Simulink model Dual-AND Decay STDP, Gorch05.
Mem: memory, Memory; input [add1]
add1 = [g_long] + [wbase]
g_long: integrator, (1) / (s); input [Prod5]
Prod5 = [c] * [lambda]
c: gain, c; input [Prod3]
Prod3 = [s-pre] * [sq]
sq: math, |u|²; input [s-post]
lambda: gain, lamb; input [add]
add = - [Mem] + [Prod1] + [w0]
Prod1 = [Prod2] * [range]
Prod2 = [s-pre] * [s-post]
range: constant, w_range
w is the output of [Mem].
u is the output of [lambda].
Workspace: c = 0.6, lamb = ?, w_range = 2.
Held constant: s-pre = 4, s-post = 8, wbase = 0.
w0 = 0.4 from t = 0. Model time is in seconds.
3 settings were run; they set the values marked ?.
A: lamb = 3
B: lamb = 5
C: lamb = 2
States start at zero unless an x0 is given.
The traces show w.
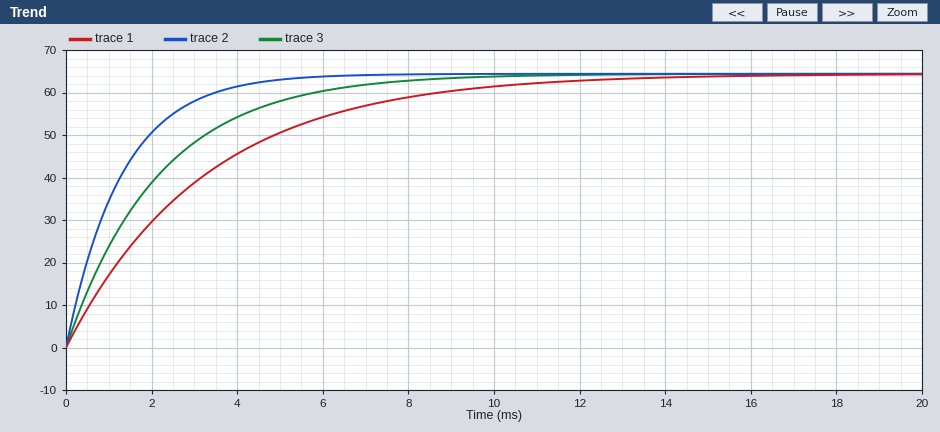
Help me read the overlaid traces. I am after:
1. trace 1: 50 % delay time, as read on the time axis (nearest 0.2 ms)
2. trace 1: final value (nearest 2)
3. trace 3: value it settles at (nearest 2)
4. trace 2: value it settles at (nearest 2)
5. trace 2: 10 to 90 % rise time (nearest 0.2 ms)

2.2 ms
64
64
64
2.8 ms
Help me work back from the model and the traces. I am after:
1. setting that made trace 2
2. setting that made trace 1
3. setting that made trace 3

B
C
A
